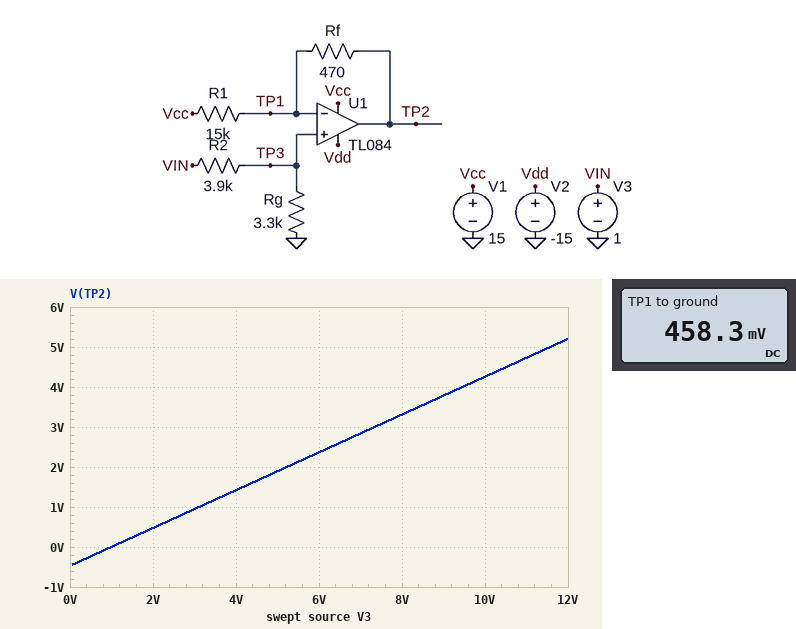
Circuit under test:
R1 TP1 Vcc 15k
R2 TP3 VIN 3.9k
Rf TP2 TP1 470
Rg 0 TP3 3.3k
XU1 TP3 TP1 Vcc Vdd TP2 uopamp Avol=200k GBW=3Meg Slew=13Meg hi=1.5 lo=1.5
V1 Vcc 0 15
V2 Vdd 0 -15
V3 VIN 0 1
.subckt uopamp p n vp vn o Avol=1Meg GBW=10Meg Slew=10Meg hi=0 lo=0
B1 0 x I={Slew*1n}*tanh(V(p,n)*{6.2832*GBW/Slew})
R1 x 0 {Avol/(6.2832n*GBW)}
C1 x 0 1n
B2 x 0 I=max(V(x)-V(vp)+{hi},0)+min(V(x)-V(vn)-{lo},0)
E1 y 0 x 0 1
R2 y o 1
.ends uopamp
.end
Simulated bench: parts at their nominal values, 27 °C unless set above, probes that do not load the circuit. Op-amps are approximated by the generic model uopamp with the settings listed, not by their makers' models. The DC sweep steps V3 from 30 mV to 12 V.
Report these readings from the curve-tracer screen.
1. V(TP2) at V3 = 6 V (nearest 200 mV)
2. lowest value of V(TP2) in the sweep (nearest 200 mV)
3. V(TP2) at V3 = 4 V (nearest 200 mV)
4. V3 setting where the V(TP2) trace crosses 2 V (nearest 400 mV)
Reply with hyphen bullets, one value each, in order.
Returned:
- 2.4 V
- -400 mV
- 1.4 V
- 5.2 V
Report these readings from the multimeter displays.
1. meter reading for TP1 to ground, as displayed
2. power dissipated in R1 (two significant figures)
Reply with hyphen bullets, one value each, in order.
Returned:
- 458.3 mV
- 14 mW
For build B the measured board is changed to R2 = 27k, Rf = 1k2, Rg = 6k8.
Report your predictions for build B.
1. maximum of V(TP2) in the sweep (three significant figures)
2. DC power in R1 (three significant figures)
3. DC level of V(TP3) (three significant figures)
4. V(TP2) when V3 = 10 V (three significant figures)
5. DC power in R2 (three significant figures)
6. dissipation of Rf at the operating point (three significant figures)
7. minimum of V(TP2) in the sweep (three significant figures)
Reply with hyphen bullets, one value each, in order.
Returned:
- 1.41 V
- 14.6 mW
- 201 mV
- 973 mV
- 23.6 µW
- 1.17 mW
- -1.19 V
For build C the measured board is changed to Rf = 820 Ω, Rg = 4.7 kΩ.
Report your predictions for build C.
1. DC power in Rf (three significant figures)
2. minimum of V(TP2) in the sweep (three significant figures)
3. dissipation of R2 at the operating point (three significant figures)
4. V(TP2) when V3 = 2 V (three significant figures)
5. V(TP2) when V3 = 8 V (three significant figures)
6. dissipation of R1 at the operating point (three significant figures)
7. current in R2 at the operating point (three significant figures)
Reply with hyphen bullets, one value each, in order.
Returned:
- 761 µW
- -803 mV
- 52.7 µW
- 333 mV
- 3.79 V
- 13.9 mW
- 116 µA
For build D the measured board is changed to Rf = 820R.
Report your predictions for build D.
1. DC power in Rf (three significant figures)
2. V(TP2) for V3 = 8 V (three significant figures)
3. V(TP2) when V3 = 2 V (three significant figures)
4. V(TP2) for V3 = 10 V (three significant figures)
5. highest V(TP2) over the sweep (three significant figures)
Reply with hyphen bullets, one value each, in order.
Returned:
- 771 µW
- 3.05 V
- 147 mV
- 4.01 V
- 4.98 V
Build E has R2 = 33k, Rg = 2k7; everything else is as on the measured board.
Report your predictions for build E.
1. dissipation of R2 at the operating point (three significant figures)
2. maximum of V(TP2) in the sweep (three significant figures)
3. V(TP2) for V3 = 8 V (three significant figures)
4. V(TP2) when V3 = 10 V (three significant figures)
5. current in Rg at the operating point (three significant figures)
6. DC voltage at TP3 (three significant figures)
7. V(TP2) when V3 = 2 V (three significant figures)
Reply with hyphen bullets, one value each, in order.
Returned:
- 25.9 µW
- 466 mV
- 154 mV
- 310 mV
- 28.0 µA
- 75.6 mV
- -314 mV
